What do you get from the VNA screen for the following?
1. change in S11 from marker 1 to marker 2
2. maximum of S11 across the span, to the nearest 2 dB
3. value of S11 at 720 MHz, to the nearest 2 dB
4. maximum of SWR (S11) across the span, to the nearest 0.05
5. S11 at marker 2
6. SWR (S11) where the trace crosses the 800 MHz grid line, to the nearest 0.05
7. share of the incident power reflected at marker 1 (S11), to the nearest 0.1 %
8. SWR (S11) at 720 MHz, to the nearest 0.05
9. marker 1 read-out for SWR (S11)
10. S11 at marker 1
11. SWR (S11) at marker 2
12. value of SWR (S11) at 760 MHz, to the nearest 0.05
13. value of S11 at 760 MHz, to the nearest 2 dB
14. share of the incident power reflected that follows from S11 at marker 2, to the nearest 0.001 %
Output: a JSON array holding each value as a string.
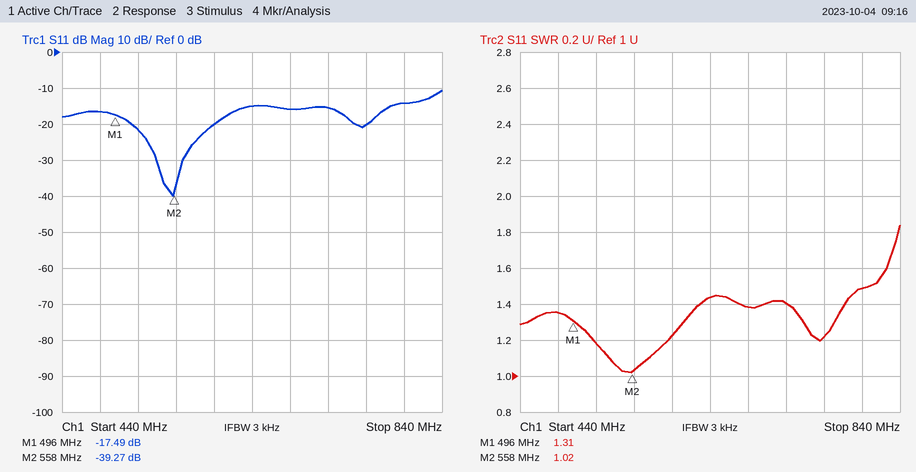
["-21.78 dB", "-10 dB", "-16 dB", "1.85", "-39.27 dB", "1.50", "1.8 %", "1.40", "1.31", "-17.49 dB", "1.02", "1.20", "-20 dB", "0.012 %"]
